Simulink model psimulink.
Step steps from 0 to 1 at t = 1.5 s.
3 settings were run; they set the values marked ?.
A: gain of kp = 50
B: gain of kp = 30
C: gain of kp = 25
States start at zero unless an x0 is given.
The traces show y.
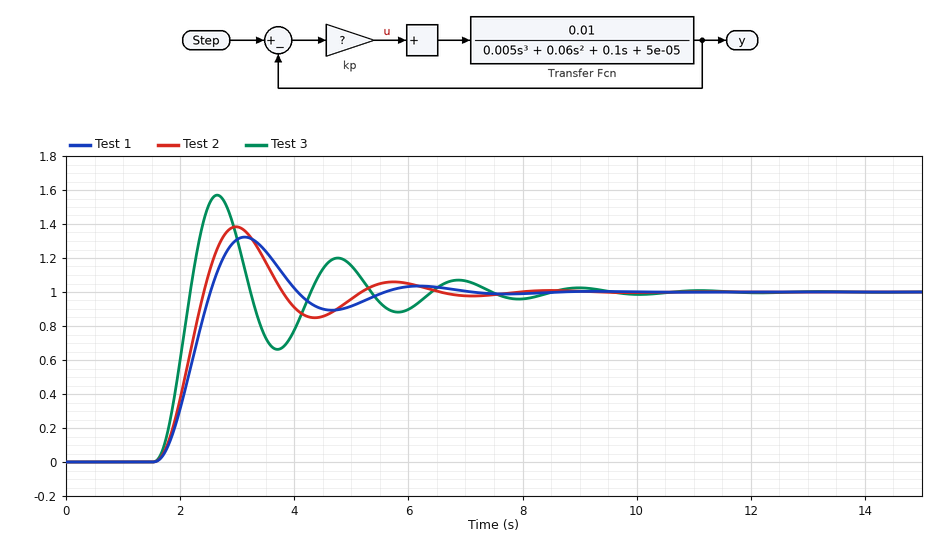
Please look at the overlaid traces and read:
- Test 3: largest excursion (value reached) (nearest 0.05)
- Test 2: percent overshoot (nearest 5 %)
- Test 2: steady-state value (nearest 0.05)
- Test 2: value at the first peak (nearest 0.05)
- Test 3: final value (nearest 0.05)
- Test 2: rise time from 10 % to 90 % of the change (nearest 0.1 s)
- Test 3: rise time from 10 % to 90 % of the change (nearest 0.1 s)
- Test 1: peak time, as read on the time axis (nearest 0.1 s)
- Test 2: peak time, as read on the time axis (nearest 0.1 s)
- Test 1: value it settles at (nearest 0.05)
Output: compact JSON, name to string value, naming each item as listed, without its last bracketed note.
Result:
{"Test 3: largest excursion (value reached)": "1.55", "Test 2: percent overshoot": "40 %", "Test 2: steady-state value": "1.00", "Test 2: value at the first peak": "1.40", "Test 3: final value": "1.00", "Test 2: rise time from 10 % to 90 % of the change": "0.6 s", "Test 3: rise time from 10 % to 90 % of the change": "0.4 s", "Test 1: peak time, as read on the time axis": "3.1 s", "Test 2: peak time, as read on the time axis": "3.0 s", "Test 1: value it settles at": "1.00"}
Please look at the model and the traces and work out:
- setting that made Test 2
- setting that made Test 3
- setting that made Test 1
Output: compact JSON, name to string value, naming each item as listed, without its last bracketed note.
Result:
{"setting that made Test 2": "B", "setting that made Test 3": "A", "setting that made Test 1": "C"}
